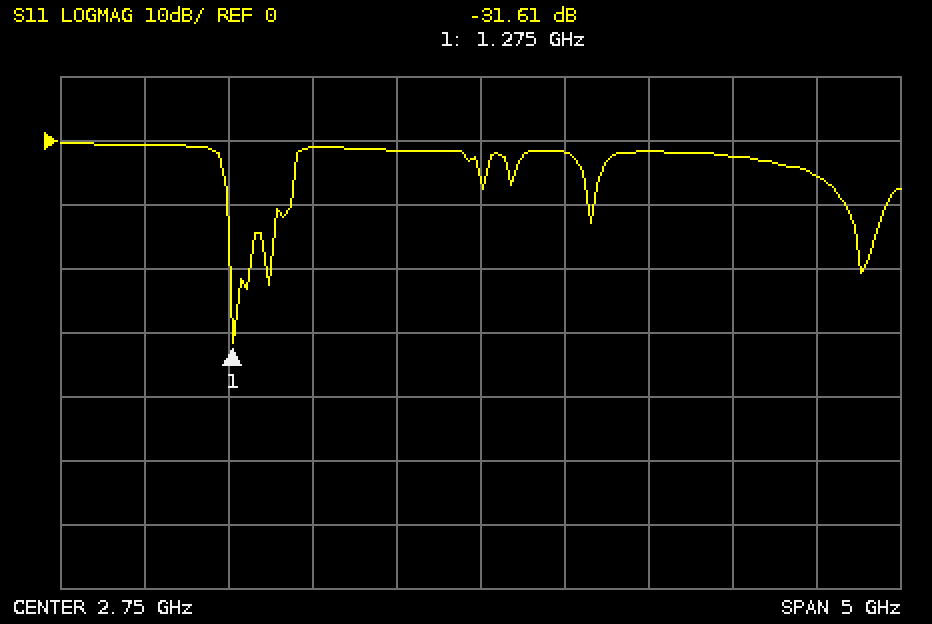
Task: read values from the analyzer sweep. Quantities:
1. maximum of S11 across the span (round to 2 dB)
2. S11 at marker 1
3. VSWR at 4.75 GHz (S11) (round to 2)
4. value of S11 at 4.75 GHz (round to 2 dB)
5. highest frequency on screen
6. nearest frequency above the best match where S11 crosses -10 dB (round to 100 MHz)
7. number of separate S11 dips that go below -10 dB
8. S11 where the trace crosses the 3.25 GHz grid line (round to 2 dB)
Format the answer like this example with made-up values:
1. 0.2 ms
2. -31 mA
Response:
1. 0 dB
2. -31.61 dB
3. 4
4. -6 dB
5. 5.25 GHz
6. 1.6 GHz
7. 4
8. -2 dB
